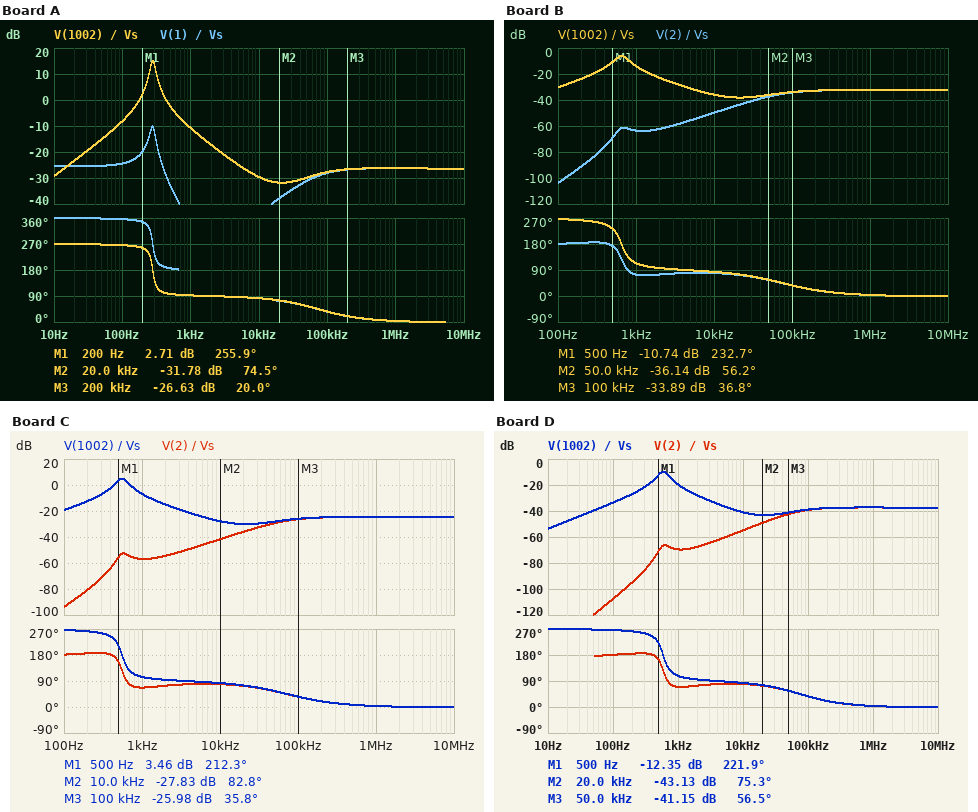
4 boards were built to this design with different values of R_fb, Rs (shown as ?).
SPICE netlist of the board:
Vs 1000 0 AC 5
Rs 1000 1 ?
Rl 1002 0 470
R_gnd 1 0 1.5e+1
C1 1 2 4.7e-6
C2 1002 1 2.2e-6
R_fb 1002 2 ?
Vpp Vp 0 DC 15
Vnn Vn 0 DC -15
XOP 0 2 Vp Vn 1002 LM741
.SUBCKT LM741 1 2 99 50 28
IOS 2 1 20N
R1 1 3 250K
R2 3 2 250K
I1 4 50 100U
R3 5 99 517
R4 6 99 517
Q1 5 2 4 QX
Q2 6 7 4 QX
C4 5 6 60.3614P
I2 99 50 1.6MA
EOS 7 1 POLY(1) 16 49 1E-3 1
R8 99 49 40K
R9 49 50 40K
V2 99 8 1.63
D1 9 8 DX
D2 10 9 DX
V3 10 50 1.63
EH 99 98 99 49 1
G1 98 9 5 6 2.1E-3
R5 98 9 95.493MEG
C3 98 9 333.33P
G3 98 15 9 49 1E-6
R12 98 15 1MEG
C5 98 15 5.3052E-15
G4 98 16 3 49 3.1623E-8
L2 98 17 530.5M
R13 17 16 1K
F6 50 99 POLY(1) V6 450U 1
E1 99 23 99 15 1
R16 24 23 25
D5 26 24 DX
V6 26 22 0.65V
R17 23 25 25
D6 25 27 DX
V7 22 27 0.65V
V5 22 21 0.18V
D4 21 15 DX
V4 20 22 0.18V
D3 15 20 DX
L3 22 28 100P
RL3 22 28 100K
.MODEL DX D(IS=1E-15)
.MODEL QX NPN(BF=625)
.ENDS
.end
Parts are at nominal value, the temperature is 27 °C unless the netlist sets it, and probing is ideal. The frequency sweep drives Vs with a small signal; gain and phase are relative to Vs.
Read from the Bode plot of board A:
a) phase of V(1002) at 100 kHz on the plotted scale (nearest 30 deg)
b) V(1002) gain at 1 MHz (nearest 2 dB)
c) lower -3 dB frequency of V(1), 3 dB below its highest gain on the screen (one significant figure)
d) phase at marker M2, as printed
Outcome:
30 deg
-26 dB
300 Hz
74.5 deg
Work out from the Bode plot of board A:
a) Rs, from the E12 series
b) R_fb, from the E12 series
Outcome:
270 Ω
2.2 kΩ
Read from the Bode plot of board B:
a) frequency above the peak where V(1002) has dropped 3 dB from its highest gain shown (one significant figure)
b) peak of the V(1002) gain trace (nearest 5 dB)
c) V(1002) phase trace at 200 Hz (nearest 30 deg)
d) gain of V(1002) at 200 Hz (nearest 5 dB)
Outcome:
800 Hz
-5 dB
270 deg
-25 dB
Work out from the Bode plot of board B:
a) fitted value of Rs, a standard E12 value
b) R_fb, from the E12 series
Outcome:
560 Ω
390 Ω
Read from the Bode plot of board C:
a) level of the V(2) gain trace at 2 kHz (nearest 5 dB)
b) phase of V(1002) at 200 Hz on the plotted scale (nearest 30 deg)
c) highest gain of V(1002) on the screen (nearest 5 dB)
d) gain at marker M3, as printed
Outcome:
-55 dB
270 deg
5 dB
-25.98 dB
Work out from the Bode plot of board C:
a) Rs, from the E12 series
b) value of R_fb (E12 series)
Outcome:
220 Ω
560 Ω
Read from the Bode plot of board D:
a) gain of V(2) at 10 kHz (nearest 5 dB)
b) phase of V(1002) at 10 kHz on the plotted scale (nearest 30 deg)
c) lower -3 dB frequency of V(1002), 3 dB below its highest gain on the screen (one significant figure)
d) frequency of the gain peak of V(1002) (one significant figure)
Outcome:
-55 dB
90 deg
500 Hz
600 Hz
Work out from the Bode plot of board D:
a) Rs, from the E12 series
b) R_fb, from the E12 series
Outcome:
1 kΩ
470 Ω
